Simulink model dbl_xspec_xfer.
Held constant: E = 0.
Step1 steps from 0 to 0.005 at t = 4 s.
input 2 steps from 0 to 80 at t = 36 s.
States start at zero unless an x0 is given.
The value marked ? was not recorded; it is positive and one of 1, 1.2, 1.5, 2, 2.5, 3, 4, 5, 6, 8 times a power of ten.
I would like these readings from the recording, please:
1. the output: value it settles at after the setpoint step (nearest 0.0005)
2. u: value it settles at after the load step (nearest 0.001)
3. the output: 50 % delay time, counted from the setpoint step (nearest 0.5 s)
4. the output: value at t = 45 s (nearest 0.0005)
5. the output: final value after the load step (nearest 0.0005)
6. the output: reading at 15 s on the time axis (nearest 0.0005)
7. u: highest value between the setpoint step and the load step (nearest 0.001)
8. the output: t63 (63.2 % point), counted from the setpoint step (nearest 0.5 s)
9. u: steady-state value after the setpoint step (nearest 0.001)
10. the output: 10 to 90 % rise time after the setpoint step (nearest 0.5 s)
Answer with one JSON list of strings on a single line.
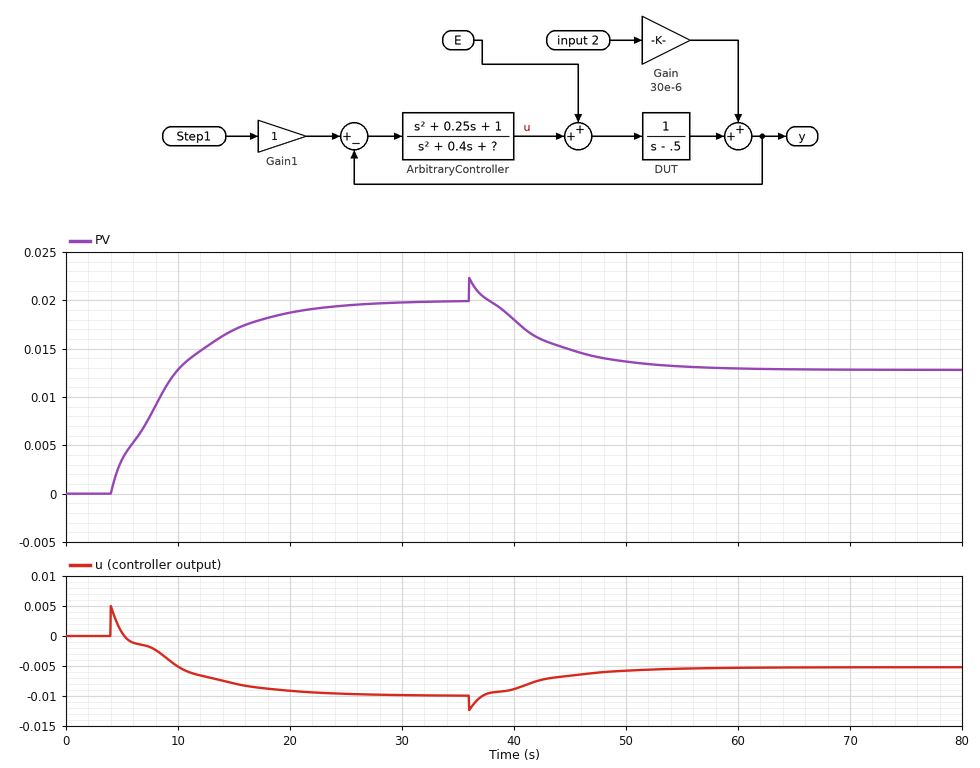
["0.0200", "-0.005", "4.5 s", "0.0150", "0.0130", "0.0170", "0.005", "6.0 s", "-0.010", "13.0 s"]
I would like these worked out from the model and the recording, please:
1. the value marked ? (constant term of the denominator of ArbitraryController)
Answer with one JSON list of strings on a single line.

["1.5"]
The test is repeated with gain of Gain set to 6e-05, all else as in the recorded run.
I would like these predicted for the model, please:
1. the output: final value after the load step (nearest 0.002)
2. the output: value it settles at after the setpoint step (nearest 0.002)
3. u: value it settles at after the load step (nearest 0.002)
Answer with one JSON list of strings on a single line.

["0.006", "0.020", "0.000"]
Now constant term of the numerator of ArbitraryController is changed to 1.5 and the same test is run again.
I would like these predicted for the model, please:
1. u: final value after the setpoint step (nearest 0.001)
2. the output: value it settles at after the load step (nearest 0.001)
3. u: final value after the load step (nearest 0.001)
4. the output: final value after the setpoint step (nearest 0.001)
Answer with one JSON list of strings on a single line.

["-0.005", "0.008", "-0.003", "0.010"]
